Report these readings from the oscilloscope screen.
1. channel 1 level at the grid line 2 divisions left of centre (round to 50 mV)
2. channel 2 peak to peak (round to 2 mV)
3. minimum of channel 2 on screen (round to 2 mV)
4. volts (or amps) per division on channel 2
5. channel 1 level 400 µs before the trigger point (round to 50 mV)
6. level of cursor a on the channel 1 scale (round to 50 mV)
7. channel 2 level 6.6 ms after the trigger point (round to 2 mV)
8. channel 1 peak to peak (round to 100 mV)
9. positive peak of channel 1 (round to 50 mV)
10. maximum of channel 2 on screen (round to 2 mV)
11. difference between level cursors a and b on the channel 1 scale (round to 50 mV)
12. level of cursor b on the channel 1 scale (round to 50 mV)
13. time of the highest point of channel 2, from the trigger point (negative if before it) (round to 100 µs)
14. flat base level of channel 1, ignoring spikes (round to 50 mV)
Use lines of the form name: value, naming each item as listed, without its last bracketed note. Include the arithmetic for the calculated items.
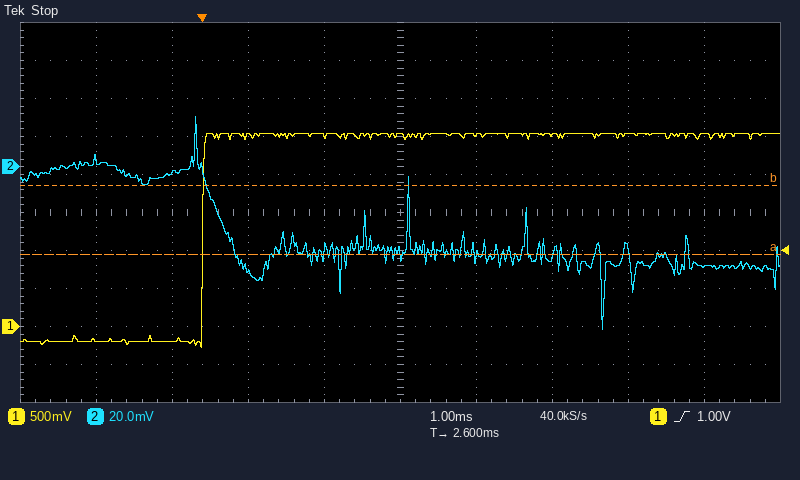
channel 1 level at the grid line 2 divisions left of centre: 2.50 V
channel 2 peak to peak: 26 mV − (-86 mV) = 112 mV
minimum of channel 2 on screen: -86 mV
volts (or amps) per division on channel 2: 20 mV
channel 1 level 400 µs before the trigger point: -200 mV
level of cursor a on the channel 1 scale: 950 mV
channel 2 level 6.6 ms after the trigger point: -52 mV
channel 1 peak to peak: 2.80 V
positive peak of channel 1: 2.55 V
maximum of channel 2 on screen: 26 mV
difference between level cursors a and b on the channel 1 scale: 900 mV
level of cursor b on the channel 1 scale: 1.85 V
time of the highest point of channel 2, from the trigger point (negative if before it): -100 µs
flat base level of channel 1, ignoring spikes: -200 mV
